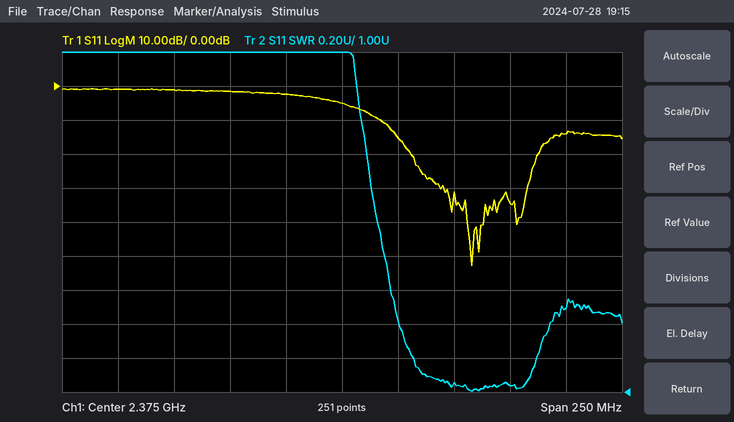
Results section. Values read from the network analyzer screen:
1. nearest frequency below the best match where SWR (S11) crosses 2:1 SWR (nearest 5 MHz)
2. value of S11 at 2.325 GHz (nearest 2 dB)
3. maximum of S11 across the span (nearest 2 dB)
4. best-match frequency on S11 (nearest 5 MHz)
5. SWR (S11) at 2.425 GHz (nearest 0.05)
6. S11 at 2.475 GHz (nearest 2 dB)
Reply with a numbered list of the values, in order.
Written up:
1. 2.390 GHz
2. -2 dB
3. 0 dB
4. 2.435 GHz
5. 1.05
6. -14 dB
